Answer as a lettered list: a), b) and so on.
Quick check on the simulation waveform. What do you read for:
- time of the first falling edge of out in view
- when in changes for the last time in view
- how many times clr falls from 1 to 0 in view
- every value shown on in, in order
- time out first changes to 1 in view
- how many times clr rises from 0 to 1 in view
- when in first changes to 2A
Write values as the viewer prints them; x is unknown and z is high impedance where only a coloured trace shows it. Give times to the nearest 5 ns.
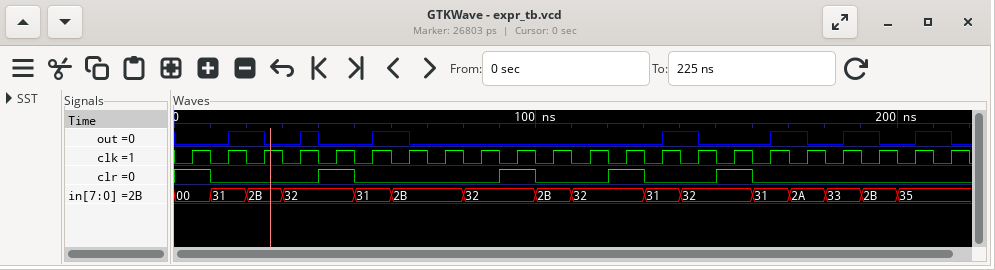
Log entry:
a) 25 ns
b) 200 ns
c) 5
d) 00, 31, 2B, 32, 31, 2B, 32, 2B, 32, 31, 32, 31, 2A, 33, 2B, 35
e) 15 ns
f) 4
g) 170 ns
